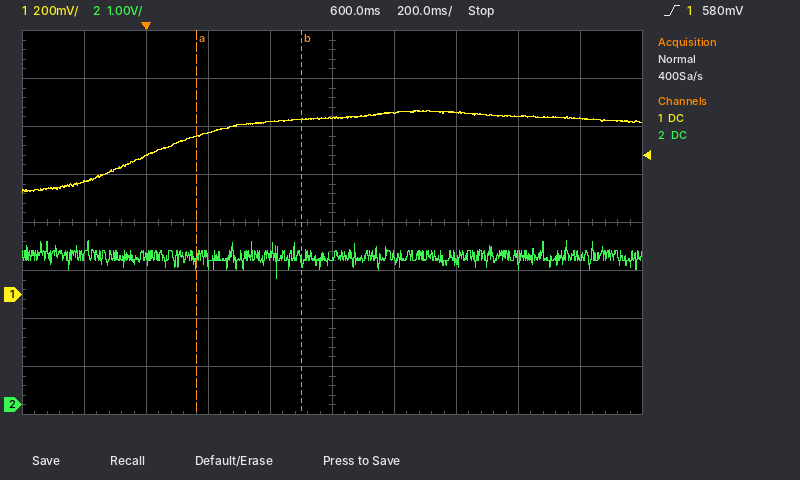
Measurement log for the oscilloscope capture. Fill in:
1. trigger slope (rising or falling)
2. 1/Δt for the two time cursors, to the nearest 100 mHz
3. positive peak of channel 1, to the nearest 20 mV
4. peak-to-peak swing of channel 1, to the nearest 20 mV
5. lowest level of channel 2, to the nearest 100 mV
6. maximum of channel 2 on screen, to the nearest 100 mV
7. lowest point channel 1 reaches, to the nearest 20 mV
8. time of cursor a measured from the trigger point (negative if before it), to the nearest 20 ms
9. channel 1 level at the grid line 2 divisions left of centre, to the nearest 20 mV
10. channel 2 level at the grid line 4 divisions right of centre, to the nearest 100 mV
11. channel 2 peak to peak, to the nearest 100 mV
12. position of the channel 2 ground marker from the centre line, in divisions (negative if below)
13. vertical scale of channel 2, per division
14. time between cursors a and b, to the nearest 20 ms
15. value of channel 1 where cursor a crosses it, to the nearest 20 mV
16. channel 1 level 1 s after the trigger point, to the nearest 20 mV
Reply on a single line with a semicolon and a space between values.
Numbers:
rising; 2.9 Hz; 760 mV; 340 mV; 2.6 V; 3.4 V; 420 mV; +160 ms; 680 mV; 3.1 V; 800 mV; -3.8 div; 1 V; 340 ms; 660 mV; 760 mV
